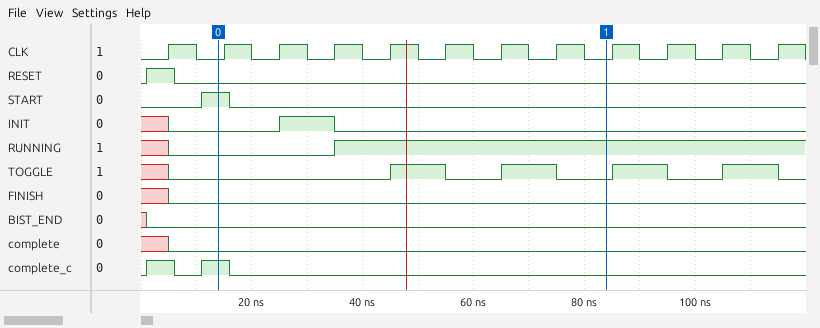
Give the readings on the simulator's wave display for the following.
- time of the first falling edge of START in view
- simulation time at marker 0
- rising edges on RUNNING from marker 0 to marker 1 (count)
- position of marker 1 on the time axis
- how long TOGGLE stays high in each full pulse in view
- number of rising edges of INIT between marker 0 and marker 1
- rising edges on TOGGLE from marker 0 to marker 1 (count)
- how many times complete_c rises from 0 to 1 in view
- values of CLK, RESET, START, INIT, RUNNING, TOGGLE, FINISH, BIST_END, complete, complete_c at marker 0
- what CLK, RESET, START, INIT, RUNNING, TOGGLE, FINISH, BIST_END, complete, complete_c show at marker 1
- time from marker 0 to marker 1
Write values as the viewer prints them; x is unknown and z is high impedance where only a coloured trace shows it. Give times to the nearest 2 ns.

16 ns
14 ns
1
84 ns
10 ns, 10 ns, 10 ns, 10 ns
1
2
2
CLK=0, RESET=0, START=1, INIT=0, RUNNING=0, TOGGLE=0, FINISH=0, BIST_END=0, complete=0, complete_c=1
CLK=0, RESET=0, START=0, INIT=0, RUNNING=1, TOGGLE=0, FINISH=0, BIST_END=0, complete=0, complete_c=0
70 ns
